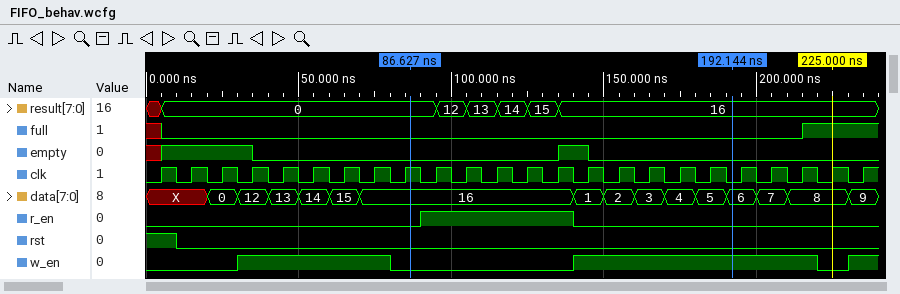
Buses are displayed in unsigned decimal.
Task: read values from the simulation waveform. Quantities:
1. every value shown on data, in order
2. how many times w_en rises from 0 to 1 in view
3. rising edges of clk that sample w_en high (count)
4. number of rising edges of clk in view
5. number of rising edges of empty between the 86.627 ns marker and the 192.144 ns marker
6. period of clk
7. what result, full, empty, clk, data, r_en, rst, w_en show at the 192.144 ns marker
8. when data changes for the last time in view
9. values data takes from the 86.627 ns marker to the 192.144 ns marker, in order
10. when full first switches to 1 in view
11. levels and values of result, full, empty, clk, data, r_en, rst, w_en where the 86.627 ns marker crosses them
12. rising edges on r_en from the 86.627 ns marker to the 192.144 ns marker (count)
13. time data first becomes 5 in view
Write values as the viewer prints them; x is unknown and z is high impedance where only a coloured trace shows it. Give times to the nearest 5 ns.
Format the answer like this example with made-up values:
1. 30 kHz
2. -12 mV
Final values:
1. X, 0, 12, 13, 14, 15, 16, 1, 2, 3, 4, 5, 6, 7, 8, 9
2. 3
3. 14
4. 24
5. 1
6. 10 ns
7. result=16, full=0, empty=0, clk=0, data=6, r_en=0, rst=0, w_en=1
8. 230 ns
9. 16, 1, 2, 3, 4, 5, 6
10. 215 ns
11. result=0, full=0, empty=0, clk=1, data=16, r_en=0, rst=0, w_en=0
12. 1
13. 180 ns
